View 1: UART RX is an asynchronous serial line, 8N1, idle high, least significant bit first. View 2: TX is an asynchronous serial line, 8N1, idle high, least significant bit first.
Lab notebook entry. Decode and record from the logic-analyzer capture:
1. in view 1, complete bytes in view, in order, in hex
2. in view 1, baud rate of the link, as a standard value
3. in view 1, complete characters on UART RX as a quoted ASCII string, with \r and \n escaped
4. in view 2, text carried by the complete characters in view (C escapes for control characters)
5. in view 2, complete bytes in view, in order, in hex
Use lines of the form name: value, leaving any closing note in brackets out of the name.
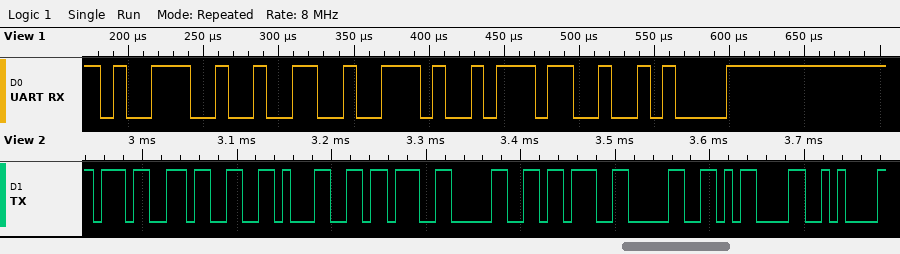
in view 1, complete bytes in view, in order, in hex: 39 32 2E 37 0A
in view 1, baud rate of the link, as a standard value: 115200 baud
in view 1, complete characters on UART RX as a quoted ASCII string, with \r and \n escaped: "92.7\n"
in view 2, text carried by the complete characters in view: "731;0;0\r\n"
in view 2, complete bytes in view, in order, in hex: 0x37 0x33 0x31 0x3B 0x30 0x3B 0x30 0x0D 0x0A
